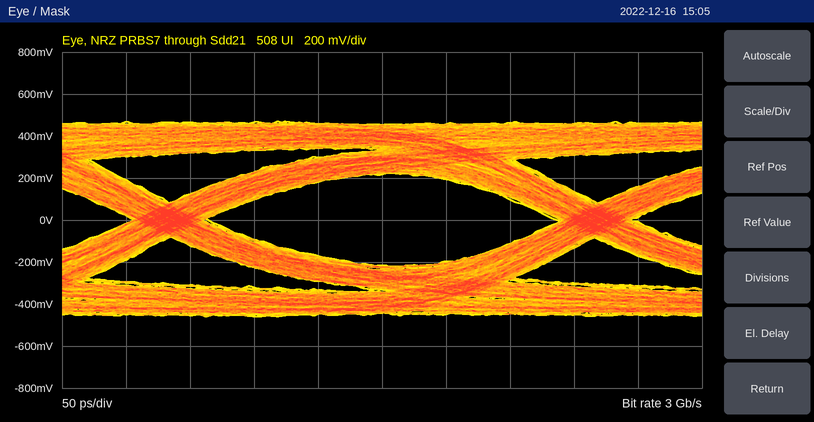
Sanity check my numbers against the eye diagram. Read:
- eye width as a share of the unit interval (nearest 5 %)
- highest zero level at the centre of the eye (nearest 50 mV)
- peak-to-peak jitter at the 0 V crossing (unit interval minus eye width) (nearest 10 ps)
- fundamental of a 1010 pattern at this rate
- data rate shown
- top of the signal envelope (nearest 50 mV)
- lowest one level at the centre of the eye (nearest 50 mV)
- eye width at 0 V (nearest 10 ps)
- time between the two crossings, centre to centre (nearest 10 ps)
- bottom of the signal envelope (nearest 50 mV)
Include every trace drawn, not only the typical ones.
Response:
80 %
-200 mV
60 ps
1.5 GHz
3 Gb/s
450 mV
200 mV
270 ps
330 ps
-450 mV
